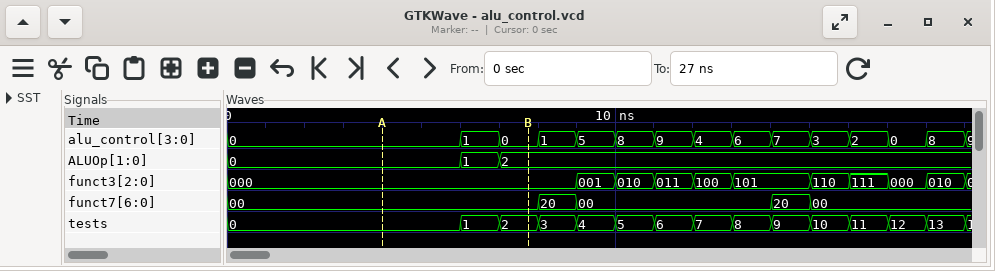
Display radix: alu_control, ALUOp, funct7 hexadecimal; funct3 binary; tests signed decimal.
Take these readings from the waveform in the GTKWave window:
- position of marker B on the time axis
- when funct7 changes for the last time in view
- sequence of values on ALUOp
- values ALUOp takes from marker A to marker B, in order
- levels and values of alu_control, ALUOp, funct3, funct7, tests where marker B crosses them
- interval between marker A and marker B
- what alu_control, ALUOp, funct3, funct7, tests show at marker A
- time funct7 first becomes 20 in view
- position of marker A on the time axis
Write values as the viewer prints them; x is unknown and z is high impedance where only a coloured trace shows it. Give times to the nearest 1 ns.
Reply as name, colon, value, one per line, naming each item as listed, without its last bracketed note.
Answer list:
position of marker B on the time axis: 8 ns
when funct7 changes for the last time in view: 15 ns
sequence of values on ALUOp: 0, 1, 2
values ALUOp takes from marker A to marker B, in order: 0, 1, 2
levels and values of alu_control, ALUOp, funct3, funct7, tests where marker B crosses them: alu_control=0, ALUOp=2, funct3=000, funct7=00, tests=2
interval between marker A and marker B: 4 ns
what alu_control, ALUOp, funct3, funct7, tests show at marker A: alu_control=0, ALUOp=0, funct3=000, funct7=00, tests=0
time funct7 first becomes 20 in view: 8 ns
position of marker A on the time axis: 4 ns
